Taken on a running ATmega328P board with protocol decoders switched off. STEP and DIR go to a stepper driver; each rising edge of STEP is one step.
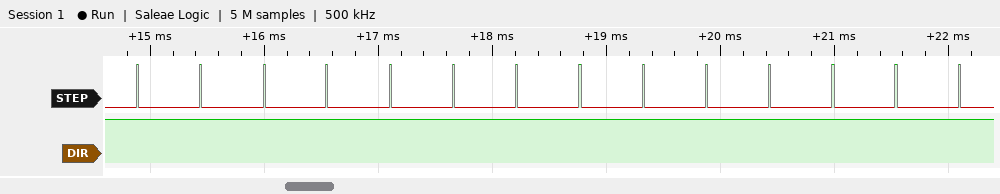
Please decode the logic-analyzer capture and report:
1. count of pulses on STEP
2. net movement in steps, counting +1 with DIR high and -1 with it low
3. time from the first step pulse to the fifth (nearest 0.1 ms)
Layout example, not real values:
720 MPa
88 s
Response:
14
+14
2.2 ms
